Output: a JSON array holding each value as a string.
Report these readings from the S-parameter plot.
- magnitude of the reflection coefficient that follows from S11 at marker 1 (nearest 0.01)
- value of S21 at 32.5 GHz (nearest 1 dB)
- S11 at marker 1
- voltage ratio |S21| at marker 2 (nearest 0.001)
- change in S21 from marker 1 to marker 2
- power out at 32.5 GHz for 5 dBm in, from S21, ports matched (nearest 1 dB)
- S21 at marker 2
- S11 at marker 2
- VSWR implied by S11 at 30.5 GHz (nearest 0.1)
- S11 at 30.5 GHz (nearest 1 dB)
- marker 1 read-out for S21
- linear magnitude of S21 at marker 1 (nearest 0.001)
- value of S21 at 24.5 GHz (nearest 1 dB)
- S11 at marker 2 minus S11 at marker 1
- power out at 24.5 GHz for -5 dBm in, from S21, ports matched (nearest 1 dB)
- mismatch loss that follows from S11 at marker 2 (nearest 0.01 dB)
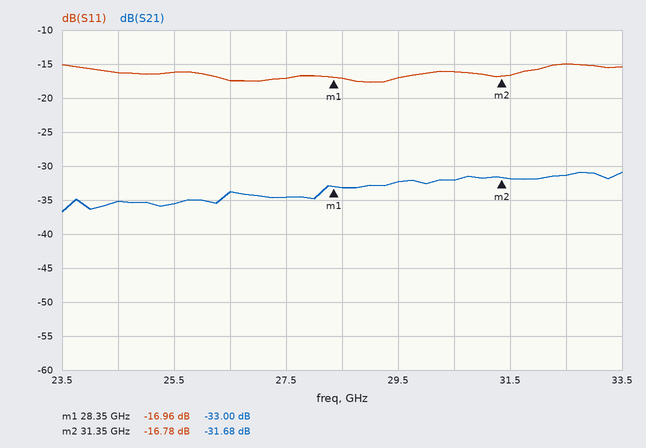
["0.14", "-31 dB", "-16.96 dB", "0.026", "1.32 dB", "-26 dBm", "-31.68 dB", "-16.78 dB", "1.4", "-16 dB", "-33.00 dB", "0.022", "-35 dB", "0.18 dB", "-40 dBm", "0.09 dB"]
